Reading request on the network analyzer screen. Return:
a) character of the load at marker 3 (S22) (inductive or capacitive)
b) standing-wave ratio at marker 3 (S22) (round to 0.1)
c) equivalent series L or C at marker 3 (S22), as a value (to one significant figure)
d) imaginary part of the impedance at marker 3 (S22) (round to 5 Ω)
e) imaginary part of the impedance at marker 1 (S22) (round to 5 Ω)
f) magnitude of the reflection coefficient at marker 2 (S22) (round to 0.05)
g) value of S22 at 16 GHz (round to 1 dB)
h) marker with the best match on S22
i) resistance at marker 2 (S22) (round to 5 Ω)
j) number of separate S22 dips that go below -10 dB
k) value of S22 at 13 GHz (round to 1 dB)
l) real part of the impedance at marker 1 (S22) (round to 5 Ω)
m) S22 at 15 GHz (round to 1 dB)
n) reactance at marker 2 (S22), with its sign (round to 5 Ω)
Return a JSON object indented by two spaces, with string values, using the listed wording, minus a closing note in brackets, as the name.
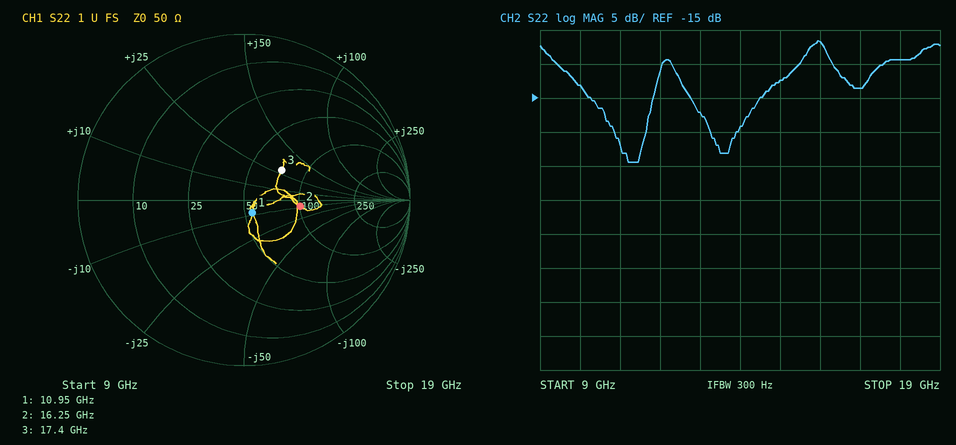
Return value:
{
  "character of the load at marker 3 (S22)": "inductive",
  "standing-wave ratio at marker 3 (S22)": "1.8",
  "equivalent series L or C at marker 3 (S22), as a value": "300 pH",
  "imaginary part of the impedance at marker 3 (S22)": "+30 Ω",
  "imaginary part of the impedance at marker 1 (S22)": "-10 Ω",
  "magnitude of the reflection coefficient at marker 2 (S22)": "0.35",
  "value of S22 at 16 GHz": "-7 dB",
  "marker with the best match on S22": "marker 1",
  "resistance at marker 2 (S22)": "100 Ω",
  "number of separate S22 dips that go below -10 dB": "3",
  "value of S22 at 13 GHz": "-17 dB",
  "real part of the impedance at marker 1 (S22)": "55 Ω",
  "S22 at 15 GHz": "-12 dB",
  "reactance at marker 2 (S22), with its sign": "-10 Ω"
}
